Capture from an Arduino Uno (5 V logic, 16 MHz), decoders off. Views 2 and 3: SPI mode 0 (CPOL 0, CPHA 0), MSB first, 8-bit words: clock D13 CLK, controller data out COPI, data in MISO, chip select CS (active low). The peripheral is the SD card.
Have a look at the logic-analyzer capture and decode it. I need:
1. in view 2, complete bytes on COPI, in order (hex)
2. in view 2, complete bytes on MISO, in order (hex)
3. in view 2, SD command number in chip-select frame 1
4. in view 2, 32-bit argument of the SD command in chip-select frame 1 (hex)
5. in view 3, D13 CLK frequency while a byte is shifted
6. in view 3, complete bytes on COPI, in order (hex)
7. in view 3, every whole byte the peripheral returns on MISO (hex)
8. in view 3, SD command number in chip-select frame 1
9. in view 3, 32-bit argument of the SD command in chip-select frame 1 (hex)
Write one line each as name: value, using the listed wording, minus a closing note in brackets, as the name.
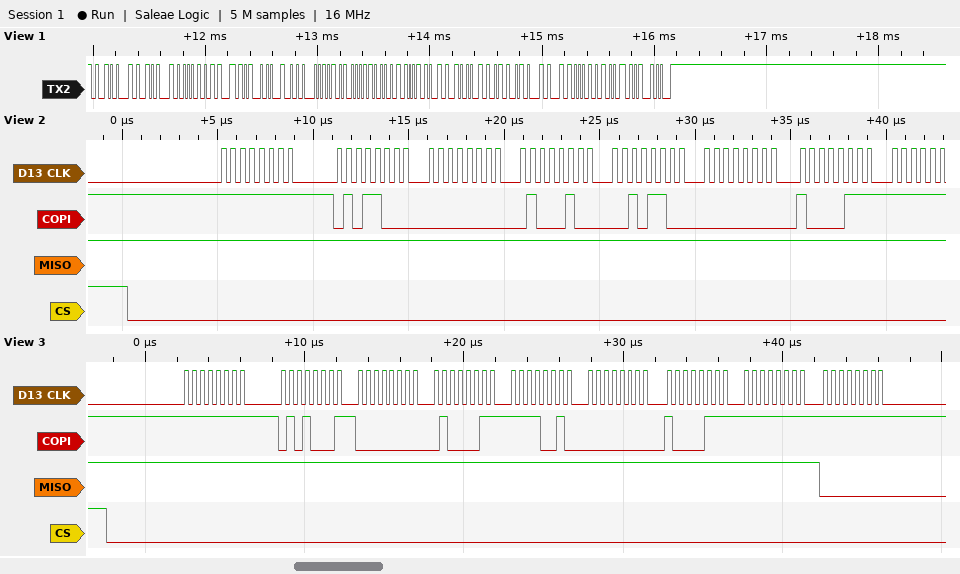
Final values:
in view 2, complete bytes on COPI, in order: FF 58 00 44 2C 00 87
in view 2, complete bytes on MISO, in order: FF FF FF FF FF FF FF
in view 2, SD command number in chip-select frame 1: CMD24
in view 2, 32-bit argument of the SD command in chip-select frame 1: 0x00442C00
in view 3, D13 CLK frequency while a byte is shifted: 2 MHz
in view 3, complete bytes on COPI, in order: FF 51 00 43 F2 00 87 FF FF
in view 3, every whole byte the peripheral returns on MISO: FF FF FF FF FF FF FF FF 00
in view 3, SD command number in chip-select frame 1: CMD17
in view 3, 32-bit argument of the SD command in chip-select frame 1: 0x0043F200
